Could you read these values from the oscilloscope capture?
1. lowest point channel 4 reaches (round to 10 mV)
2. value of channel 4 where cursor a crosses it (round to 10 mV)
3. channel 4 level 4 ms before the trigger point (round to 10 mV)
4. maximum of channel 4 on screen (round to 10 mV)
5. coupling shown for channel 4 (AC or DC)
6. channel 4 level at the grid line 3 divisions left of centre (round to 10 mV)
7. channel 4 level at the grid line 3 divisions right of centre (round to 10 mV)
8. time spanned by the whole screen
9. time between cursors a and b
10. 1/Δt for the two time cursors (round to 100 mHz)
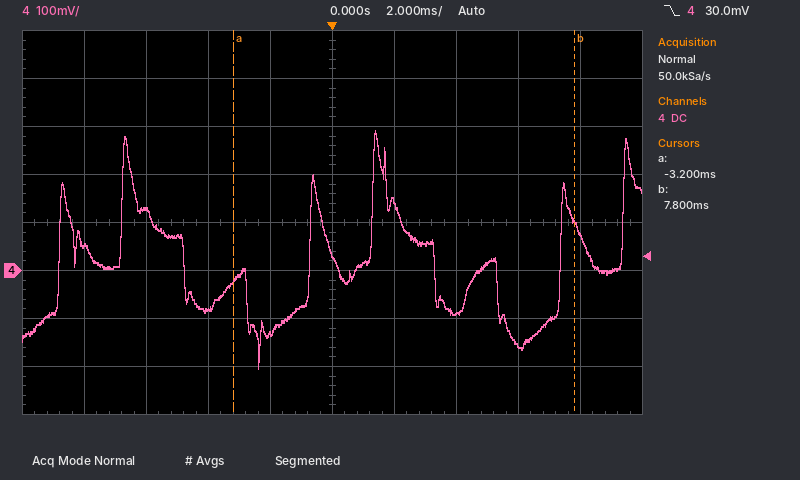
-200 mV
-20 mV
-80 mV
290 mV
DC
130 mV
-150 mV
20 ms
11.0 ms
90.9 Hz
